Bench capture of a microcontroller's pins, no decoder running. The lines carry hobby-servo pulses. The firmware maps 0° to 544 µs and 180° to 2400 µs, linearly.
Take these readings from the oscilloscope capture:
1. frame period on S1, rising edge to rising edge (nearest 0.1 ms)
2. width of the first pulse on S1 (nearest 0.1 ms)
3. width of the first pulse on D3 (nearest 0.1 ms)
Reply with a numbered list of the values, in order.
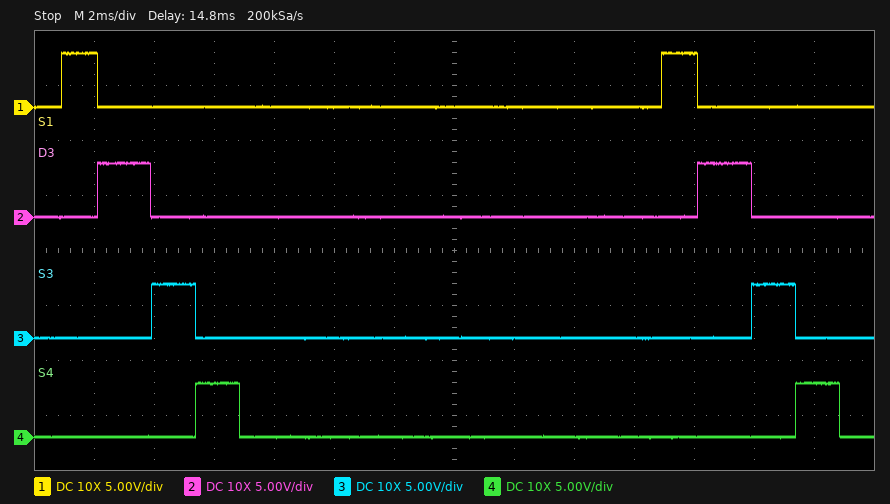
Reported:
1. 20.0 ms
2. 1.2 ms
3. 1.8 ms
